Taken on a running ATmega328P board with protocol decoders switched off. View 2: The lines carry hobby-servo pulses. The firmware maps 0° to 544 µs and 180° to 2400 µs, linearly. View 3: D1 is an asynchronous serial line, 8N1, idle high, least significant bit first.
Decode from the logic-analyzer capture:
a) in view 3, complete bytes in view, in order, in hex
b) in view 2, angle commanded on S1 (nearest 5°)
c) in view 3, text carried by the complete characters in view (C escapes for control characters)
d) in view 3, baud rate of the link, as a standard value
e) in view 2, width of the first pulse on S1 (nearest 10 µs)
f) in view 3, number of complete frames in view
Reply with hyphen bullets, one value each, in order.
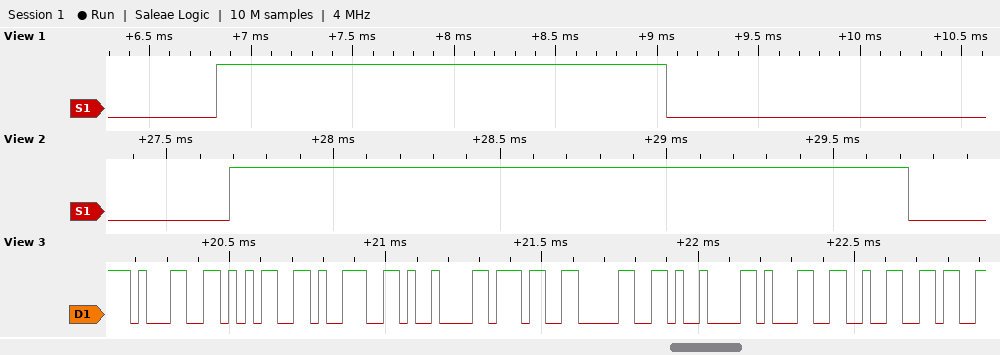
- 0x31 0x35 0x39 0x09 0x37 0x30 0x09 0x31 0x32
- 145°
- "159\t70\t12"
- 38400 baud
- 2040 µs
- 9
